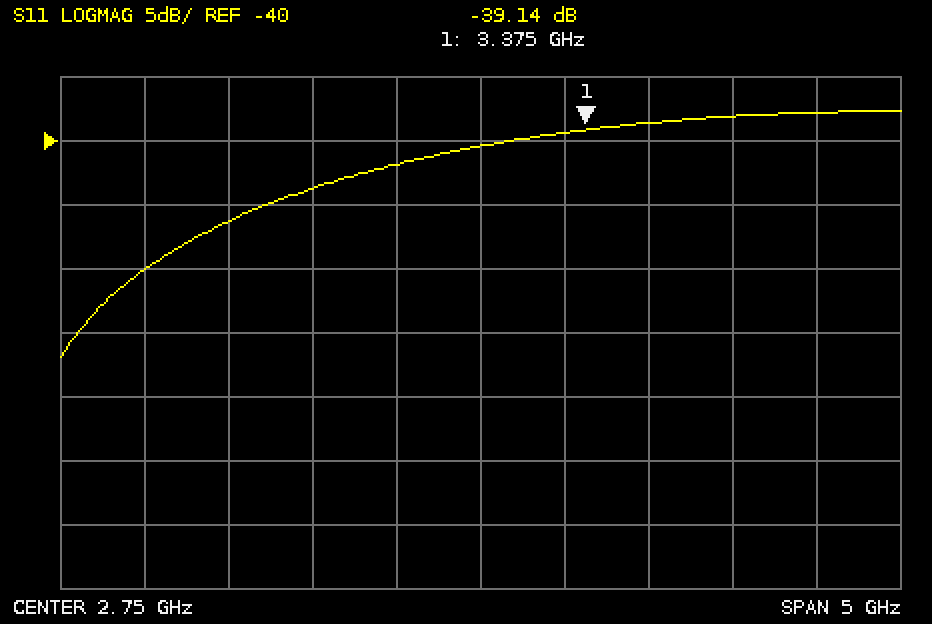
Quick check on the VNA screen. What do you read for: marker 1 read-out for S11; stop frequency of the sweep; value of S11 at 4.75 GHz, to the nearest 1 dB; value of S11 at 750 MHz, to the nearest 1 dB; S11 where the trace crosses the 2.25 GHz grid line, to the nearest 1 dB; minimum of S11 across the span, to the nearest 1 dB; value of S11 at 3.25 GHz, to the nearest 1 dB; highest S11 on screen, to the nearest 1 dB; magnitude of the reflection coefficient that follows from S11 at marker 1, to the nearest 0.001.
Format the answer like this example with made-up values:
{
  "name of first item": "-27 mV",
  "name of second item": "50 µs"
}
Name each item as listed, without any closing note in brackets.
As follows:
{
  "marker 1 read-out for S11": "-39.14 dB",
  "stop frequency of the sweep": "5.25 GHz",
  "value of S11 at 4.75 GHz, to the nearest 1 dB": "-38 dB",
  "value of S11 at 750 MHz, to the nearest 1 dB": "-50 dB",
  "S11 where the trace crosses the 2.25 GHz grid line, to the nearest 1 dB": "-42 dB",
  "minimum of S11 across the span, to the nearest 1 dB": "-57 dB",
  "value of S11 at 3.25 GHz, to the nearest 1 dB": "-39 dB",
  "highest S11 on screen, to the nearest 1 dB": "-38 dB",
  "magnitude of the reflection coefficient that follows from S11 at marker 1, to the nearest 0.001": "0.011"
}
